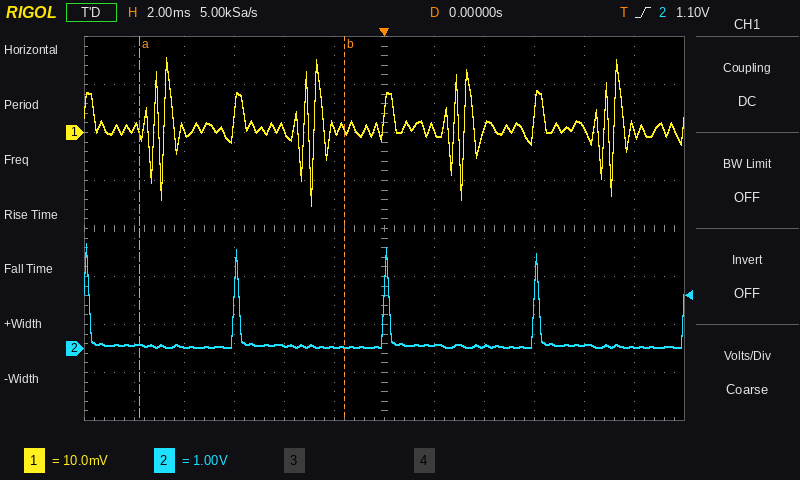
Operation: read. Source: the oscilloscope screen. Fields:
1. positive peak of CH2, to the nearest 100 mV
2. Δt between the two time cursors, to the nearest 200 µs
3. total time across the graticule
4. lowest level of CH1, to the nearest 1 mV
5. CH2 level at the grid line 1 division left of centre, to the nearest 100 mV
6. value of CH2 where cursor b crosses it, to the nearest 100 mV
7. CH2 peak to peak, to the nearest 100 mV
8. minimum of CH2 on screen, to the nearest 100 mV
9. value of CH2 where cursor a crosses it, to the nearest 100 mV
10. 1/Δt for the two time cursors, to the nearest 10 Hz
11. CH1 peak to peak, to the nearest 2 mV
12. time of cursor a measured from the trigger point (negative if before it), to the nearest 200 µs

2.2 V
8.2 ms
24 ms
-15 mV
0.0 V
0.0 V
2.2 V
0.0 V
100 mV
120 Hz
30 mV
-9.8 ms
